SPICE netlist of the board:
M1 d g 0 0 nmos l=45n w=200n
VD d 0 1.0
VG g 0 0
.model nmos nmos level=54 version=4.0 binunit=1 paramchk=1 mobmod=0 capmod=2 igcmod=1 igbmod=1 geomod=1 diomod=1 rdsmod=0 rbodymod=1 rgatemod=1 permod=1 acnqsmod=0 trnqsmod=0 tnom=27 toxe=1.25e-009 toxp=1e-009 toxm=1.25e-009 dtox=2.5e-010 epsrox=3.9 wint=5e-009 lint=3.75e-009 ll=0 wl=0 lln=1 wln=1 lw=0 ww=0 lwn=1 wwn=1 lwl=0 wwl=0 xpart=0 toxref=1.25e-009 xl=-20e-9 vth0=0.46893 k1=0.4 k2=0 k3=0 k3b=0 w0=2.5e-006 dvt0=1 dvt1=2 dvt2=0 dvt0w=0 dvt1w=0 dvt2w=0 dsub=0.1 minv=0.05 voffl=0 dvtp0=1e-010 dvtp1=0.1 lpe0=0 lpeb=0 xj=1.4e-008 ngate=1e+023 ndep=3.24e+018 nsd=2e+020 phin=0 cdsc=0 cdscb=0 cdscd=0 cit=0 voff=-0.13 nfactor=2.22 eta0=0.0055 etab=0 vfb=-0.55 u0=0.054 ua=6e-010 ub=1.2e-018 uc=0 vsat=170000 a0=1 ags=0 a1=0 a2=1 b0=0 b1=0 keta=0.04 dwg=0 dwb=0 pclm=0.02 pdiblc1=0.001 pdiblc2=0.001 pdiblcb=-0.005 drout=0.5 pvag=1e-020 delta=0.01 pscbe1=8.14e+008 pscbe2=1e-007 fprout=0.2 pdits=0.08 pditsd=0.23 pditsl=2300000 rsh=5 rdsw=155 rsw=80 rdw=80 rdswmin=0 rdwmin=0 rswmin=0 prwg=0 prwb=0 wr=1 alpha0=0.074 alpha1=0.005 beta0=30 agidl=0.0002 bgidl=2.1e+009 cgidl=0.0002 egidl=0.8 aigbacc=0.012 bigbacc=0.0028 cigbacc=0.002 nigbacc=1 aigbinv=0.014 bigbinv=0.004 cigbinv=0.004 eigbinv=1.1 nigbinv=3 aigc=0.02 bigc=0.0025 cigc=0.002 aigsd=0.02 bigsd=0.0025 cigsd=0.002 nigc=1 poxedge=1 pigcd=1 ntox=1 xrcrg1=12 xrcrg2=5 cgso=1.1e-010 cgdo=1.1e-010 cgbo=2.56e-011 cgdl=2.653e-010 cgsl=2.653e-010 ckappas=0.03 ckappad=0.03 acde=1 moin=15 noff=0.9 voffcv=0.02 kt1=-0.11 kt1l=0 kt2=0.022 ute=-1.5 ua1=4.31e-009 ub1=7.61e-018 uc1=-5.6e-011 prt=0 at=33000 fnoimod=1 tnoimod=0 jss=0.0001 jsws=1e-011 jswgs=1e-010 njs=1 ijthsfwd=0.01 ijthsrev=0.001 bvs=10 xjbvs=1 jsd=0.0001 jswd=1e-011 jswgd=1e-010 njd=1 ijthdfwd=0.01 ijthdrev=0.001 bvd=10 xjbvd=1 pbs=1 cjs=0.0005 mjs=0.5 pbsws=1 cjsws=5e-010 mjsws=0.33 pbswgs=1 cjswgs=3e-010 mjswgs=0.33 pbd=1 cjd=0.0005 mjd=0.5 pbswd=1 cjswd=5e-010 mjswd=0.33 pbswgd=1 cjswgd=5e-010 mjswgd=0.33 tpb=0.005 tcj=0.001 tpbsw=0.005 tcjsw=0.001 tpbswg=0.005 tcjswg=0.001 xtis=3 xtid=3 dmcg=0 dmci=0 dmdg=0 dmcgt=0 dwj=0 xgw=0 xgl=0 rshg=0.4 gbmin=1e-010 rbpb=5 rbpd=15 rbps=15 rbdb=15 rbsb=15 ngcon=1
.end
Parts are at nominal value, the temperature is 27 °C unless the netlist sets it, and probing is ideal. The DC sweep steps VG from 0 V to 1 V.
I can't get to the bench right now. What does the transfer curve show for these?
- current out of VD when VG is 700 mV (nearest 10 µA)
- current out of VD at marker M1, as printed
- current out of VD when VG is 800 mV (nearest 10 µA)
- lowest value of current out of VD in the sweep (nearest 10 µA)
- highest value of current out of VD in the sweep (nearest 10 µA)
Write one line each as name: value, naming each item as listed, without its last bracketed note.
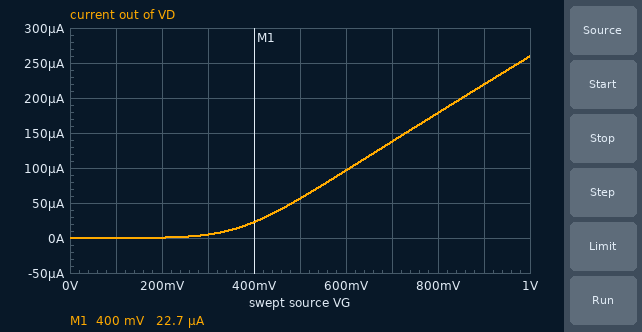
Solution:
current out of VD when VG is 700 mV: 140 µA
current out of VD at marker M1, as printed: 22.7 µA
current out of VD when VG is 800 mV: 180 µA
lowest value of current out of VD in the sweep: 0 A
highest value of current out of VD in the sweep: 260 µA
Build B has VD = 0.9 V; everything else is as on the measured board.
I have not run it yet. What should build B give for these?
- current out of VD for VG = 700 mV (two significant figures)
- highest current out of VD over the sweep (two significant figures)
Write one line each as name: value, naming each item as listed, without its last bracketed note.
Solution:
current out of VD for VG = 700 mV: 130 µA
highest current out of VD over the sweep: 250 µA
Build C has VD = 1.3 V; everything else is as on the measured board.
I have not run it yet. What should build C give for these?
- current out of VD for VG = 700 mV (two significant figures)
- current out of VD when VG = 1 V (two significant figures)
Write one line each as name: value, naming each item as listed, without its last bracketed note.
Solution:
current out of VD for VG = 700 mV: 160 µA
current out of VD when VG = 1 V: 280 µA
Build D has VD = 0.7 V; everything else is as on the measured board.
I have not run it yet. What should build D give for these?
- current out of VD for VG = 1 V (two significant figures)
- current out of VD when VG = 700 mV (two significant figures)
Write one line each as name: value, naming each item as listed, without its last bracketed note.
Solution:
current out of VD for VG = 1 V: 240 µA
current out of VD when VG = 700 mV: 120 µA
